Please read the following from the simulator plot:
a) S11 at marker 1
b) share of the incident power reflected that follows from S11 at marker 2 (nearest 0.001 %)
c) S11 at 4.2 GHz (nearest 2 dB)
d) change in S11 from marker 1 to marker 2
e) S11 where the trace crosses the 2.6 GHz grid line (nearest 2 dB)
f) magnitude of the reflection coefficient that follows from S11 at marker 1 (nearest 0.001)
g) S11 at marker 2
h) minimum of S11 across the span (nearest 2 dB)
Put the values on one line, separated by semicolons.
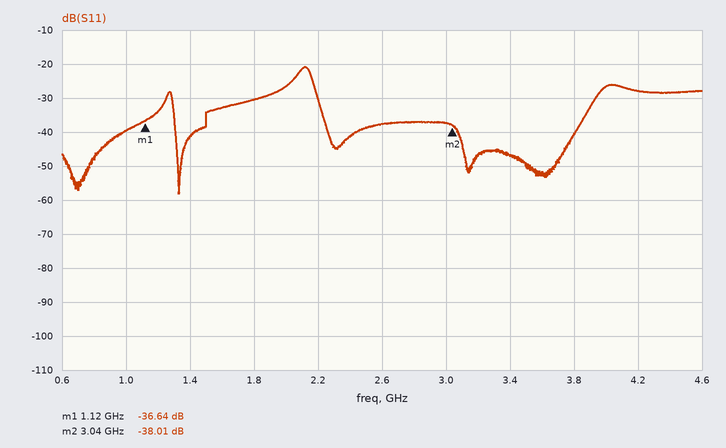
-36.64 dB; 0.016 %; -28 dB; -1.37 dB; -38 dB; 0.015; -38.01 dB; -58 dB
